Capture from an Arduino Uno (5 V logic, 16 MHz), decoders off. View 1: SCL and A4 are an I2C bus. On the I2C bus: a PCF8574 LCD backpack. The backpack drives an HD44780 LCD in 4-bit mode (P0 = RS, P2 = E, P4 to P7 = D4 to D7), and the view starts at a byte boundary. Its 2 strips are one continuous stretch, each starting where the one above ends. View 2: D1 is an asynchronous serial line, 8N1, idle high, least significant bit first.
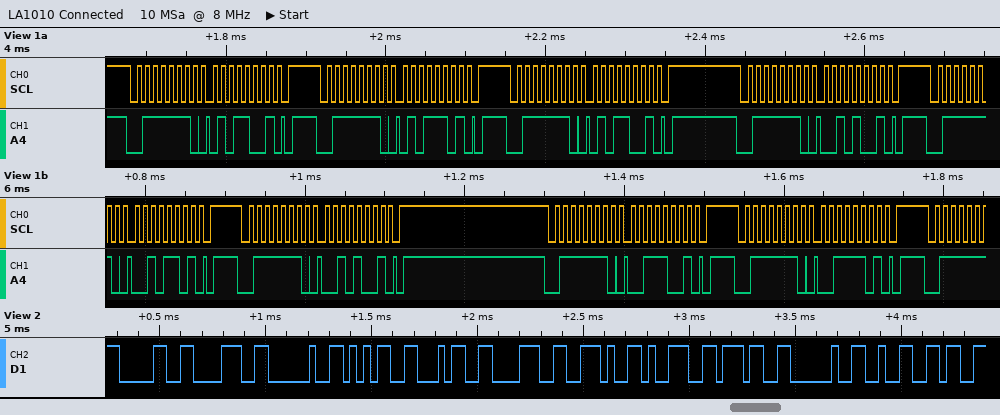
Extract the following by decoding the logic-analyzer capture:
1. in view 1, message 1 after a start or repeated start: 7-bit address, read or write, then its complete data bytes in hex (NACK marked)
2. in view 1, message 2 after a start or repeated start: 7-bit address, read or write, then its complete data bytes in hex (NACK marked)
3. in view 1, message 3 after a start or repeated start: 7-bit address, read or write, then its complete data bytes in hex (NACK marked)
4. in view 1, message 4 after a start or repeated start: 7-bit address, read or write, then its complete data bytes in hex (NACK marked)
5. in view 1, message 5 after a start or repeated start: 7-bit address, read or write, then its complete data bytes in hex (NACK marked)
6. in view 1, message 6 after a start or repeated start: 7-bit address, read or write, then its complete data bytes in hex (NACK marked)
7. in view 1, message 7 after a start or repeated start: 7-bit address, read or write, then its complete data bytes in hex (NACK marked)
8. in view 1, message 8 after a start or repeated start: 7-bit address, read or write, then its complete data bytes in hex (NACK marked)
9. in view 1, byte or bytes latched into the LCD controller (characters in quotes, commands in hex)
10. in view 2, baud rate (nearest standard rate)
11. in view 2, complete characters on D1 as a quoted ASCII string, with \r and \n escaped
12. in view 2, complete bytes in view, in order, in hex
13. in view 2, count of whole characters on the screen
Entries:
0x3F write: 59
0x3F write: 5D
0x3F write: 59
0x3F write: 29
0x3F write: 2D
0x3F write: 29
0x3F write: 39
0x3F write: 3D
'R'
31250 baud
"08 548.97 2"
30 38 20 35 34 38 2E 39 37 20 32
11
